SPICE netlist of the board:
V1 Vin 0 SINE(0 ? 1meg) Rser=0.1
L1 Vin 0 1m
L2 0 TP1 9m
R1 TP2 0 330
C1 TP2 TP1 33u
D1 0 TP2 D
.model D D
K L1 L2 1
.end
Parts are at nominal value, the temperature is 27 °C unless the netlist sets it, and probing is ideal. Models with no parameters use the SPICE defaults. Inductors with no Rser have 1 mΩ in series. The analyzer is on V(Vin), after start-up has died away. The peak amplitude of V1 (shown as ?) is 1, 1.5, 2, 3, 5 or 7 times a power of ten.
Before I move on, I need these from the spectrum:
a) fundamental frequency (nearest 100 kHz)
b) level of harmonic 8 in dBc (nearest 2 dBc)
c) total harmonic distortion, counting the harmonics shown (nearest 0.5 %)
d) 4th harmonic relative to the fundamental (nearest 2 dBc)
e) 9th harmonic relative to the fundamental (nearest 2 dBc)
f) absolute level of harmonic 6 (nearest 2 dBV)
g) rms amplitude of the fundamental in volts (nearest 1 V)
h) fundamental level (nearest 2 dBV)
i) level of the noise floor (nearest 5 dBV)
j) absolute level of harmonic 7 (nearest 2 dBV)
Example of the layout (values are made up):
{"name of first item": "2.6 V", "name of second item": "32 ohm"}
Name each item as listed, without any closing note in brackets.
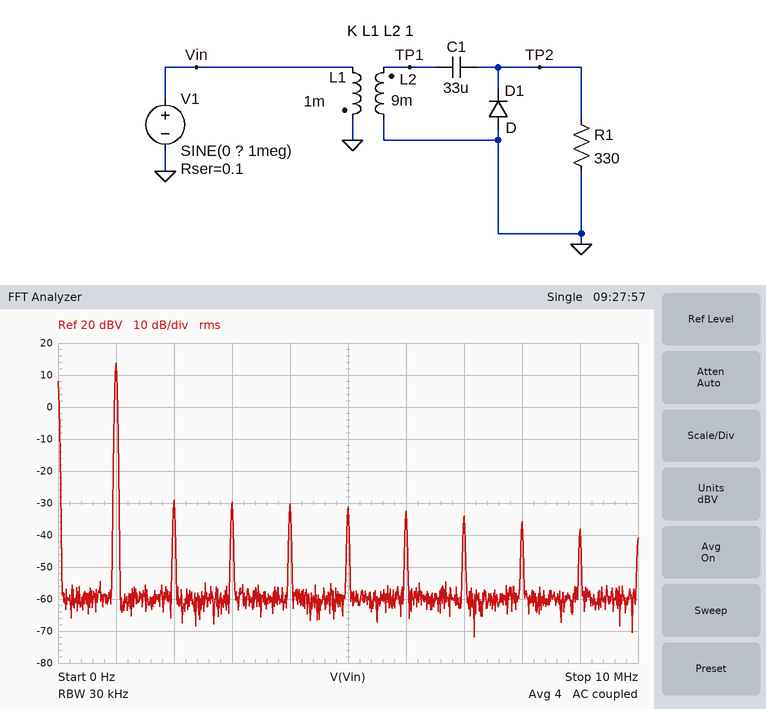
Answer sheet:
{"fundamental frequency": "1.0 MHz", "level of harmonic 8 in dBc": "-50 dBc", "total harmonic distortion, counting the harmonics shown": "1.5 %", "4th harmonic relative to the fundamental": "-44 dBc", "9th harmonic relative to the fundamental": "-52 dBc", "absolute level of harmonic 6": "-32 dBV", "rms amplitude of the fundamental in volts": "5 V", "fundamental level": "14 dBV", "level of the noise floor": "-60 dBV", "absolute level of harmonic 7": "-34 dBV"}
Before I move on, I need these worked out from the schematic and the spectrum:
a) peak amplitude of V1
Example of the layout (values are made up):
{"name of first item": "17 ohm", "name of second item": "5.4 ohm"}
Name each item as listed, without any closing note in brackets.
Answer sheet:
{"peak amplitude of V1": "7 V"}
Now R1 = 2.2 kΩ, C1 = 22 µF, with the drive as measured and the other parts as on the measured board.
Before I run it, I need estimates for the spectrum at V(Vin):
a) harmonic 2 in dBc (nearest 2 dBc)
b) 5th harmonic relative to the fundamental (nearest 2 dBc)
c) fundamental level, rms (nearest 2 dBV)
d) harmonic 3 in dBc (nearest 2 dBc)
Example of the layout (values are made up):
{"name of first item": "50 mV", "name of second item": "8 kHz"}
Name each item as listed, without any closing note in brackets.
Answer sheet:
{"harmonic 2 in dBc": "-54 dBc", "5th harmonic relative to the fundamental": "-56 dBc", "fundamental level, rms": "14 dBV", "harmonic 3 in dBc": "-54 dBc"}
